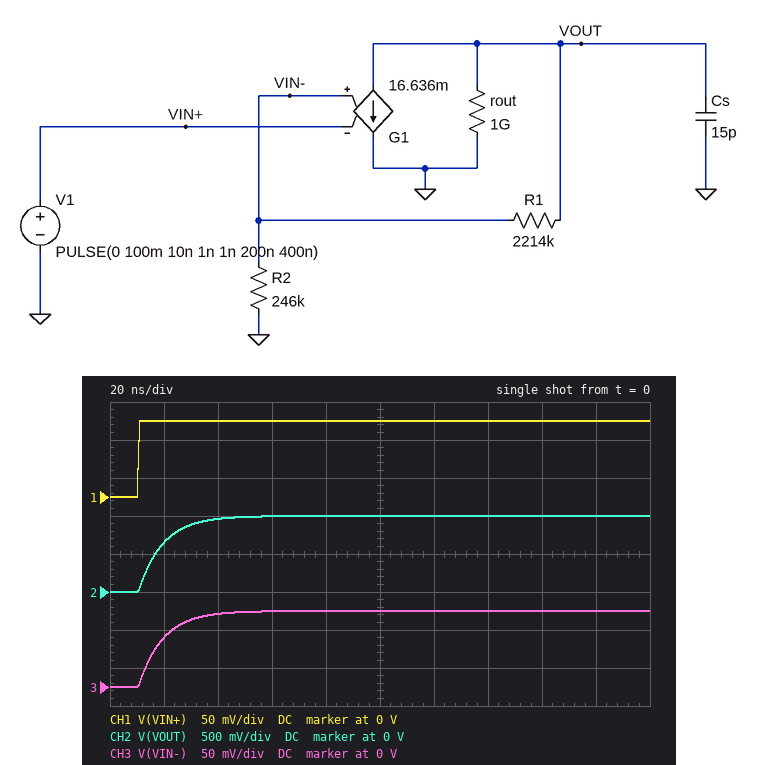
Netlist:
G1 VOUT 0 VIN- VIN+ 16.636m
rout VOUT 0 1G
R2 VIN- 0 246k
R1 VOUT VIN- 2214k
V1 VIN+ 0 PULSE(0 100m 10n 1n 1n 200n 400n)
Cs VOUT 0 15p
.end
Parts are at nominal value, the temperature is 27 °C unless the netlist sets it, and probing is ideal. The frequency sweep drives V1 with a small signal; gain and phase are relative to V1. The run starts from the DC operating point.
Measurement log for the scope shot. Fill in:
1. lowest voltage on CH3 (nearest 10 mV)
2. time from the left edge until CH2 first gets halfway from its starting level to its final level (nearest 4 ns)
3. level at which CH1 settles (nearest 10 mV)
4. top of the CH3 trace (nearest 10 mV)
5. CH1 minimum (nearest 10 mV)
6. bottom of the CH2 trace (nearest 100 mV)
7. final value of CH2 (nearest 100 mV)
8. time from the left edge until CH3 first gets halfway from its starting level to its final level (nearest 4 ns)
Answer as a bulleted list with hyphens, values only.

- 0 V
- 16 ns
- 100 mV
- 100 mV
- 0 V
- 0 V
- 1.0 V
- 16 ns
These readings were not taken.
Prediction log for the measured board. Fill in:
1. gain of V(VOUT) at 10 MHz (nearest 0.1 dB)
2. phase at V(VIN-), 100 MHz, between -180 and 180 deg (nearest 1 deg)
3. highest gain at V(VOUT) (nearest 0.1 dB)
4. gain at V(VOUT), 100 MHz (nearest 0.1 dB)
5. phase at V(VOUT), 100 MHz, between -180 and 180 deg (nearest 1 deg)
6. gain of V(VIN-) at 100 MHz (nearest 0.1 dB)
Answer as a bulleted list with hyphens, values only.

- 18.8 dB
- -80 deg
- 20.0 dB
- 4.8 dB
- -80 deg
- -15.2 dB
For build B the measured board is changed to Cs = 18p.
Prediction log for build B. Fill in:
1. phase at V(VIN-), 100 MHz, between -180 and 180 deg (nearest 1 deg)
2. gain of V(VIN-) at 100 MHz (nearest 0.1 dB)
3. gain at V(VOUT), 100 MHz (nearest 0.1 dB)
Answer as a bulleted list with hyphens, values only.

- -82 deg
- -16.7 dB
- 3.3 dB
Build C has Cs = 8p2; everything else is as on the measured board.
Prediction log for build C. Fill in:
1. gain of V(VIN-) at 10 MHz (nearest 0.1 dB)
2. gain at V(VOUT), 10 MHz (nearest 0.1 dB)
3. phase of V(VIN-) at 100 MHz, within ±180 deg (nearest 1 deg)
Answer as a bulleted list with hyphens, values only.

- -0.4 dB
- 19.6 dB
- -72 deg
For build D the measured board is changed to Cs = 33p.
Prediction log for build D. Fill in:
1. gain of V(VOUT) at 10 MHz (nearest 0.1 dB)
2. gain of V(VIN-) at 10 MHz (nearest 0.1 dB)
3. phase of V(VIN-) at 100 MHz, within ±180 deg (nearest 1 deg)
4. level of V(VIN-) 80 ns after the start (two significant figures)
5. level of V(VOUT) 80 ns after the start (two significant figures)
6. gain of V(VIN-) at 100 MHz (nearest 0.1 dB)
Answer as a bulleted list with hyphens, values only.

- 15.9 dB
- -4.1 dB
- -85 deg
- 97 mV
- 970 mV
- -21.9 dB
